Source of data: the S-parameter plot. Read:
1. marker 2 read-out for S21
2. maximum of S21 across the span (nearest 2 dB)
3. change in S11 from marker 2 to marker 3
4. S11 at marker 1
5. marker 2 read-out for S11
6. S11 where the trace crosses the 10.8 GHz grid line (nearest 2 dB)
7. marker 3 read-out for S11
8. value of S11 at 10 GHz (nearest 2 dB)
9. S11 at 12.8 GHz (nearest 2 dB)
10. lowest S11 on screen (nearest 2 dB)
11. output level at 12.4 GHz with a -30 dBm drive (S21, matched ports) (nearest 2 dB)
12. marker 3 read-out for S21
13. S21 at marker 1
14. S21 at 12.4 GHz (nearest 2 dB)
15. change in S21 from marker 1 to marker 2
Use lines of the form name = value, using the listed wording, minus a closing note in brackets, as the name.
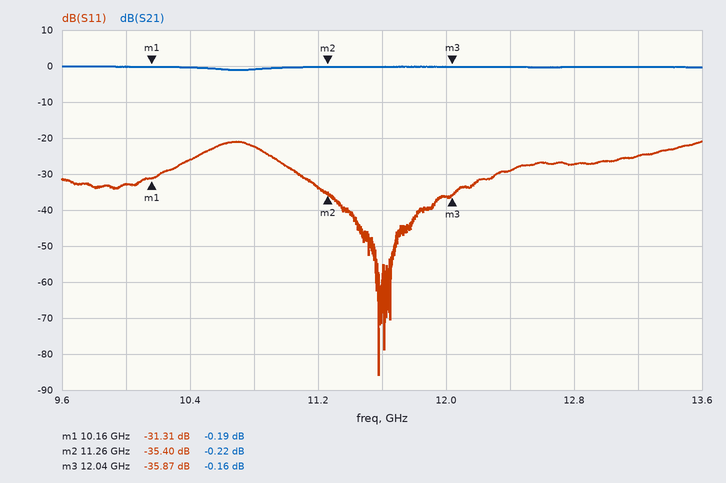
marker 2 read-out for S21 = -0.22 dB
maximum of S21 across the span = 0 dB
change in S11 from marker 2 to marker 3 = -0.47 dB
S11 at marker 1 = -31.31 dB
marker 2 read-out for S11 = -35.40 dB
S11 where the trace crosses the 10.8 GHz grid line = -22 dB
marker 3 read-out for S11 = -35.87 dB
value of S11 at 10 GHz = -32 dB
S11 at 12.8 GHz = -28 dB
lowest S11 on screen = -86 dB
output level at 12.4 GHz with a -30 dBm drive (S21, matched ports) = -30 dBm
marker 3 read-out for S21 = -0.16 dB
S21 at marker 1 = -0.19 dB
S21 at 12.4 GHz = 0 dB
change in S21 from marker 1 to marker 2 = -0.03 dB
